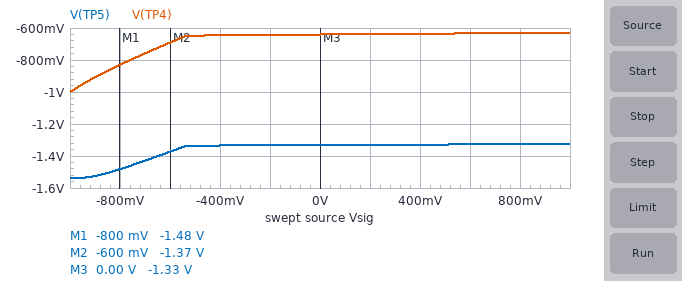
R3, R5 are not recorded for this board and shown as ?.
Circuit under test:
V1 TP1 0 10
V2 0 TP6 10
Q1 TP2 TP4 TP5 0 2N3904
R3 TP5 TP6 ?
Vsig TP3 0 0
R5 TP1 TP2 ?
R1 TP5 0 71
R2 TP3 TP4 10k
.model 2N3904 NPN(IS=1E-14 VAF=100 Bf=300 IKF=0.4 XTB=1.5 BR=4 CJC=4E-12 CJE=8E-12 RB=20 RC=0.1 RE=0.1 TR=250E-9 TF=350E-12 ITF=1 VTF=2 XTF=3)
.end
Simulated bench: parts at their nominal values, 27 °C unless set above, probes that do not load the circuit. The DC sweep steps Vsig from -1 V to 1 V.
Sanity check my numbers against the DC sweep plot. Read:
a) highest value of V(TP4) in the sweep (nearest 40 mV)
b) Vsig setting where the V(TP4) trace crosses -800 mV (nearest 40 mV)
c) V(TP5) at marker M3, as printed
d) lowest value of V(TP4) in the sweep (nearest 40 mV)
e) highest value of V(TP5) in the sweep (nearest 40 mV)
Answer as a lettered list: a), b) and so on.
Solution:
a) -640 mV
b) -760 mV
c) -1.33 V
d) -1.00 V
e) -1.32 V
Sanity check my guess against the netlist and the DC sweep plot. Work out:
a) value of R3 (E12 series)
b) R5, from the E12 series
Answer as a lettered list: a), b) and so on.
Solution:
a) 390 Ω
b) 3.3 kΩ
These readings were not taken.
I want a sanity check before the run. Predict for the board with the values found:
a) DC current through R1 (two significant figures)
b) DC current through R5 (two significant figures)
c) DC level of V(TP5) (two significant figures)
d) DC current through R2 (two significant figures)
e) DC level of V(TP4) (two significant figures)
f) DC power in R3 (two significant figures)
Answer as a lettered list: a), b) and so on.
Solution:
a) 19 mA
b) 3.4 mA
c) -1.3 V
d) 64 µA
e) -640 mV
f) 190 mW
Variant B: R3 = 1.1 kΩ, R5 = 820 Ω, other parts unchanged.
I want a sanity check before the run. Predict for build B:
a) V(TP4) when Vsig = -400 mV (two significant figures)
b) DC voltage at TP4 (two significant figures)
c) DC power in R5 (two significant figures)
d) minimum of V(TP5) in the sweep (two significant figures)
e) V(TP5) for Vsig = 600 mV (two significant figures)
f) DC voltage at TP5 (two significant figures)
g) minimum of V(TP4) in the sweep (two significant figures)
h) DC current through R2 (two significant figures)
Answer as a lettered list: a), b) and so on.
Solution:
a) -400 mV
b) -3.3 mV
c) 9.9 µW
d) -610 mV
e) -260 mV
f) -600 mV
g) -1.0 V
h) 330 nA
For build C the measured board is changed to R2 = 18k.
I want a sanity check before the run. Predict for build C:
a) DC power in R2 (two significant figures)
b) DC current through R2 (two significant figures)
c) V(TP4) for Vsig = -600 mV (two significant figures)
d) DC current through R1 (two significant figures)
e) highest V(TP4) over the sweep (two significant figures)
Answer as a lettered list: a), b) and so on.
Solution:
a) 23 µW
b) 36 µA
c) -730 mV
d) 19 mA
e) -640 mV
